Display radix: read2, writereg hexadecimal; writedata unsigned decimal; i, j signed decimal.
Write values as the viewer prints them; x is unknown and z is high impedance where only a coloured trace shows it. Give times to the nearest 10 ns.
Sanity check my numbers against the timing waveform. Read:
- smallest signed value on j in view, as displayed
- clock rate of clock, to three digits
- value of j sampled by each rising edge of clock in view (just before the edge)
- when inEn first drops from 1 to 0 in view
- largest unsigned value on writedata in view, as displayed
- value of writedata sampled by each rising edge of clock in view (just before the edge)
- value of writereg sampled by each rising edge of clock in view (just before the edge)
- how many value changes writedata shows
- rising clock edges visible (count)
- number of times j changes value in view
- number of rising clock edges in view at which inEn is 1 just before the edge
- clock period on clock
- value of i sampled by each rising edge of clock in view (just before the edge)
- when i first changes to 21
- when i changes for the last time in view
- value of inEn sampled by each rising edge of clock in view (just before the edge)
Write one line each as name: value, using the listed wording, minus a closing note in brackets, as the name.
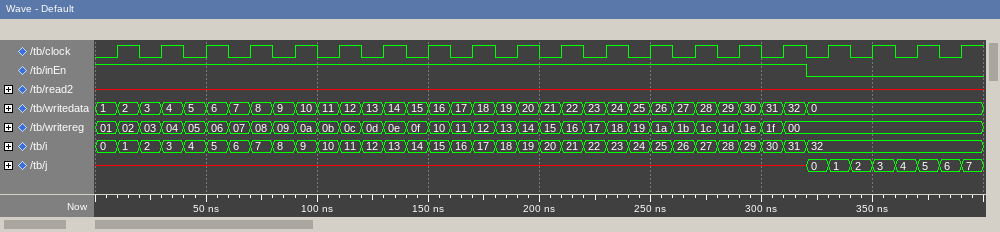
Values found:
smallest signed value on j in view, as displayed: 0
clock rate of clock, to three digits: 50.0 MHz
value of j sampled by each rising edge of clock in view: x, x, x, x, x, x, x, x, x, x, x, x, x, x, x, x, 0, 2, 4, 6
when inEn first drops from 1 to 0 in view: 320 ns
largest unsigned value on writedata in view, as displayed: 32
value of writedata sampled by each rising edge of clock in view: 1, 3, 5, 7, 9, 11, 13, 15, 17, 19, 21, 23, 25, 27, 29, 31, 0, 0, 0, 0
value of writereg sampled by each rising edge of clock in view: 01, 03, 05, 07, 09, 0b, 0d, 0f, 11, 13, 15, 17, 19, 1b, 1d, 1f, 00, 00, 00, 00
how many value changes writedata shows: 32
rising clock edges visible: 20
number of times j changes value in view: 8
number of rising clock edges in view at which inEn is 1 just before the edge: 16
clock period on clock: 20 ns
value of i sampled by each rising edge of clock in view: 0, 2, 4, 6, 8, 10, 12, 14, 16, 18, 20, 22, 24, 26, 28, 30, 32, 32, 32, 32
when i first changes to 21: 210 ns
when i changes for the last time in view: 320 ns
value of inEn sampled by each rising edge of clock in view: 1 1 1 1 1 1 1 1 1 1 1 1 1 1 1 1 0 0 0 0
